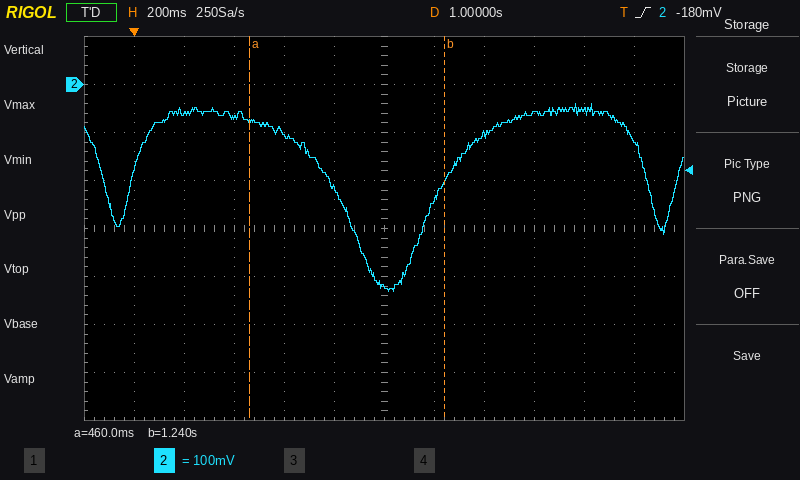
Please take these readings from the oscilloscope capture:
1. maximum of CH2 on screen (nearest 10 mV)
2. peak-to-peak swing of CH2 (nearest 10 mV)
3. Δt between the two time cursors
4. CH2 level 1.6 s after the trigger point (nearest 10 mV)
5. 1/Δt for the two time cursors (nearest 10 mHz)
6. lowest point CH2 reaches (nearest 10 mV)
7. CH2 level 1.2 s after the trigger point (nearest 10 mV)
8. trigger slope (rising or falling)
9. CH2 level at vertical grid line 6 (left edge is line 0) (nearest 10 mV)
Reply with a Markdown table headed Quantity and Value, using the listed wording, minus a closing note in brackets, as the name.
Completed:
| Quantity | Value |
|---|---|
| maximum of CH2 on screen | -40 mV |
| peak-to-peak swing of CH2 | 390 mV |
| Δt between the two time cursors | 780 ms |
| CH2 level 1.6 s after the trigger point | -60 mV |
| 1/Δt for the two time cursors | 1.28 Hz |
| lowest point CH2 reaches | -430 mV |
| CH2 level 1.2 s after the trigger point | -240 mV |
| trigger slope | rising |
| CH2 level at vertical grid line 6 (left edge is line 0) | -420 mV |
